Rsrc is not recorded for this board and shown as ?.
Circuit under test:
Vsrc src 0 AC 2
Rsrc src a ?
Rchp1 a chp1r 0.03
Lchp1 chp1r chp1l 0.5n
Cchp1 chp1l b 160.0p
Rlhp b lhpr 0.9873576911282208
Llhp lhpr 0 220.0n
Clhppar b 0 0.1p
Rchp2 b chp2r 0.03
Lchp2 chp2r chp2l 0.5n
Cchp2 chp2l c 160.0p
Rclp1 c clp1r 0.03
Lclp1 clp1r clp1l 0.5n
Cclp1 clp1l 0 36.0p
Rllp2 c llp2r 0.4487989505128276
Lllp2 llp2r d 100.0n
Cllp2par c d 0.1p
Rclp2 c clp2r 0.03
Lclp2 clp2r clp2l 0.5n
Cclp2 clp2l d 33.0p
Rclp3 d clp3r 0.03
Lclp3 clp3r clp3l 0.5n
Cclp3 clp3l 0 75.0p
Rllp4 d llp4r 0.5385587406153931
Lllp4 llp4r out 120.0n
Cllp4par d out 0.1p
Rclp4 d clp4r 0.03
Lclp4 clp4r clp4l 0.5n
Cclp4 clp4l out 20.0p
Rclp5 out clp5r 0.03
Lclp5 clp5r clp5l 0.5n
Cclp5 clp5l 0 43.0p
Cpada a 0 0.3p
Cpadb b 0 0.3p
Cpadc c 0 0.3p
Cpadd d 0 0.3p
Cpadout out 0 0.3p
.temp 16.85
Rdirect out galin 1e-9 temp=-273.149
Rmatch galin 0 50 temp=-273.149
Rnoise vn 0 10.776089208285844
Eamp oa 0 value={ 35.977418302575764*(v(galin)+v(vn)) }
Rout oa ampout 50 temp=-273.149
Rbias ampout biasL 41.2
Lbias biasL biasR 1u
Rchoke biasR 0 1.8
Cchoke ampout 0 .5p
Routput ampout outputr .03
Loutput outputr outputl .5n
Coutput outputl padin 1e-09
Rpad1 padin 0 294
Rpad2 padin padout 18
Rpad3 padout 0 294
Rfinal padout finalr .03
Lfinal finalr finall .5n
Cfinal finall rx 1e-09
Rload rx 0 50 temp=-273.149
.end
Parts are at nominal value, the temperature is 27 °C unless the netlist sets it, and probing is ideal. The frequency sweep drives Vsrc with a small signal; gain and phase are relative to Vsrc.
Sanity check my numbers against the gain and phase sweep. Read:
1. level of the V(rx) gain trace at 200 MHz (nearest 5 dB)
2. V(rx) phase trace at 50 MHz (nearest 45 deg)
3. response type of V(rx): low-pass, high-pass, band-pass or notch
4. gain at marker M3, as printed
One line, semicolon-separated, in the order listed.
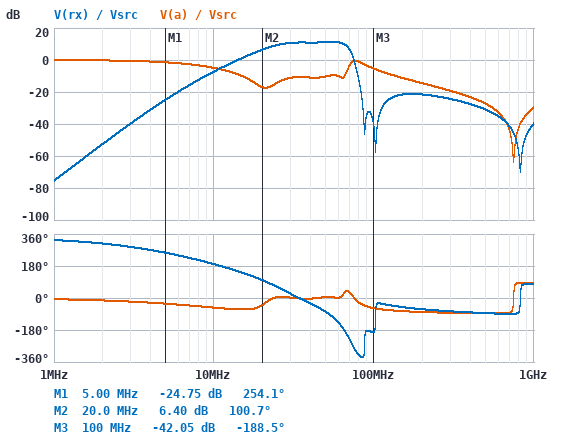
-20 dB; -90 deg; band-pass; -42.05 dB
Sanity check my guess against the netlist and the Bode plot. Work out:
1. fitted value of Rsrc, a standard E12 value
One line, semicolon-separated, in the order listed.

120 Ω
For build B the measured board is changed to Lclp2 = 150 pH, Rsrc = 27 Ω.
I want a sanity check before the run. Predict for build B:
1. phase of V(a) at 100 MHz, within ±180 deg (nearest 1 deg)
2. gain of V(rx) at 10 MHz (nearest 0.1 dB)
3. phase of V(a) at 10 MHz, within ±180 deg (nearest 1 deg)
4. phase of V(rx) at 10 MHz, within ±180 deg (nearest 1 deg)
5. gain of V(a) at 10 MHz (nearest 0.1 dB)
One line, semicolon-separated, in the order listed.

-19 deg; -2.8 dB; -18 deg; -133 deg; -0.5 dB
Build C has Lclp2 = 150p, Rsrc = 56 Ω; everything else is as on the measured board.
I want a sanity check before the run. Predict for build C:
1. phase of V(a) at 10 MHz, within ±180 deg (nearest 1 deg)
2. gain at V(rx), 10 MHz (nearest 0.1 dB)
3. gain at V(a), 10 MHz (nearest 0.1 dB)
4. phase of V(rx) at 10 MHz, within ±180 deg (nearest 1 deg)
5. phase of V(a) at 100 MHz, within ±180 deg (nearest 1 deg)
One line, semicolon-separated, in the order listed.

-33 deg; -4.0 dB; -1.7 dB; -149 deg; -36 deg
